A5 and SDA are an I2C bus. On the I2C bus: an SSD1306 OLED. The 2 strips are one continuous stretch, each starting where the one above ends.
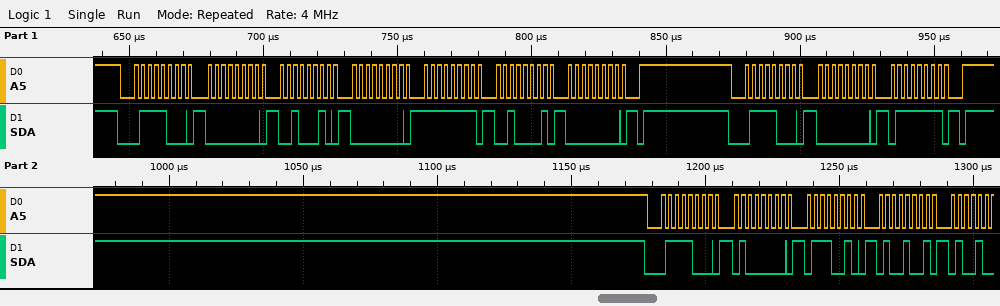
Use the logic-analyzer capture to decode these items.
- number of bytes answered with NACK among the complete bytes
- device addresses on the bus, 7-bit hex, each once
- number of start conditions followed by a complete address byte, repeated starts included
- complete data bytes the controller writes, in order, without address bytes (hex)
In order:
0
0x3C
3
00 22 00 FF 21 00 00 7F 40 72 49
